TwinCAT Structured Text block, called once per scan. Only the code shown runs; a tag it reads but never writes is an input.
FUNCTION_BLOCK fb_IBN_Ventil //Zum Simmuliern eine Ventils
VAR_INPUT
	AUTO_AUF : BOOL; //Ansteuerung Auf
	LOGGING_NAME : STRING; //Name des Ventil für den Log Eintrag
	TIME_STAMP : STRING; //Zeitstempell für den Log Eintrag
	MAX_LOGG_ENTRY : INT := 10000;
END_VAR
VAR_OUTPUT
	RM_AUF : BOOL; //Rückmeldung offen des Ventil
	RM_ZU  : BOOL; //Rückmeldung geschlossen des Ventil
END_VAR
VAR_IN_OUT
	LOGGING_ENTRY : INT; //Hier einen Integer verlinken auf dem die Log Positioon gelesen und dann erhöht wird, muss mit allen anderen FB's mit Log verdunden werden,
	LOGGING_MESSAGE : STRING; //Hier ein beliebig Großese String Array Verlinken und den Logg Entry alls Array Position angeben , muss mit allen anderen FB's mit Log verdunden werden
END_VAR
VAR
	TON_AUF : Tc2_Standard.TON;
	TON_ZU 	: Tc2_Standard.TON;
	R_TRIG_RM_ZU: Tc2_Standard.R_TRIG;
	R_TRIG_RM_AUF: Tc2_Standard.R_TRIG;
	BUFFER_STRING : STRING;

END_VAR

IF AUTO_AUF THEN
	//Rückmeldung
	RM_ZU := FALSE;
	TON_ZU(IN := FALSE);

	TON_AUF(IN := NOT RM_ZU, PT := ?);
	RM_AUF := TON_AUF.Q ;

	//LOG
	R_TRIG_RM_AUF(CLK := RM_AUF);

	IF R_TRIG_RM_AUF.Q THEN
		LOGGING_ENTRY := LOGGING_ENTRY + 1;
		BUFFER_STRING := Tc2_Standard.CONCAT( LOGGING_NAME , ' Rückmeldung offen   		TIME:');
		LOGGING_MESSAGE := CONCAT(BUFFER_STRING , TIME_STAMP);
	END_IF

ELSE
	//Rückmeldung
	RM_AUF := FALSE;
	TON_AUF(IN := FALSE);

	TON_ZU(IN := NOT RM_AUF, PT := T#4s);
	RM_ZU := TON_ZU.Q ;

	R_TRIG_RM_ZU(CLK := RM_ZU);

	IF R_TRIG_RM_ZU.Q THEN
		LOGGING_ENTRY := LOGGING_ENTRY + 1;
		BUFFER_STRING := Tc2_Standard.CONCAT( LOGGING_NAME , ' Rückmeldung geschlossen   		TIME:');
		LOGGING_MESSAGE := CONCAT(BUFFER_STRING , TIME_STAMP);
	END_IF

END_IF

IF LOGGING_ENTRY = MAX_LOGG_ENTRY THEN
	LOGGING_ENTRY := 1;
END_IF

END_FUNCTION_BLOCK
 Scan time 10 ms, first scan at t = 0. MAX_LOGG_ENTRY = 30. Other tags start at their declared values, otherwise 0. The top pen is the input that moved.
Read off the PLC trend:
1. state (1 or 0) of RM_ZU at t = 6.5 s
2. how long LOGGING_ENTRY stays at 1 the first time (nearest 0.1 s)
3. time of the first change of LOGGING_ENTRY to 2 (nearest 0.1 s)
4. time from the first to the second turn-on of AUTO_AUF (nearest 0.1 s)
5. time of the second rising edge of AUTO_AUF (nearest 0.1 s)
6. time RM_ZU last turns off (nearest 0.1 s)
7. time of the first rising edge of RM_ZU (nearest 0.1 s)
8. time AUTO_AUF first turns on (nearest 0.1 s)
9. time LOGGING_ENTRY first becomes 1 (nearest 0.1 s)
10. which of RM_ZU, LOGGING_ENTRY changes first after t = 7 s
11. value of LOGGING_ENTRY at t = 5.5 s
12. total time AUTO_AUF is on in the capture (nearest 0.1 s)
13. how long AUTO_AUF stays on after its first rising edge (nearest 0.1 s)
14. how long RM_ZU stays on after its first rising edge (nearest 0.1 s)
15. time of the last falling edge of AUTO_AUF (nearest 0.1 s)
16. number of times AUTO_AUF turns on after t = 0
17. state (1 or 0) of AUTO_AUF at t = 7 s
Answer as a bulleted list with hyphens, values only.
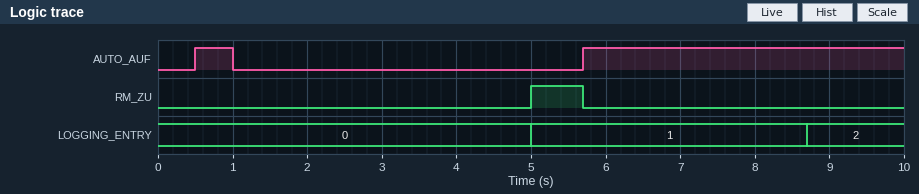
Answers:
- 0
- 3.7 s
- 8.7 s
- 5.2 s
- 5.7 s
- 5.7 s
- 5.0 s
- 0.5 s
- 5.0 s
- LOGGING_ENTRY
- 1
- 4.8 s
- 0.5 s
- 0.7 s
- 1.0 s
- 2
- 1
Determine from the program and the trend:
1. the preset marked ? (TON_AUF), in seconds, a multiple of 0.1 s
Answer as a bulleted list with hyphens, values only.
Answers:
- 3.0 s
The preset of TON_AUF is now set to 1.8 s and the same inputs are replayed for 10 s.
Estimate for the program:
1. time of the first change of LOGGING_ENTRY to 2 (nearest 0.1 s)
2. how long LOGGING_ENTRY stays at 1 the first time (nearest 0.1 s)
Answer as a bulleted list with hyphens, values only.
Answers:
- 7.5 s
- 2.5 s
